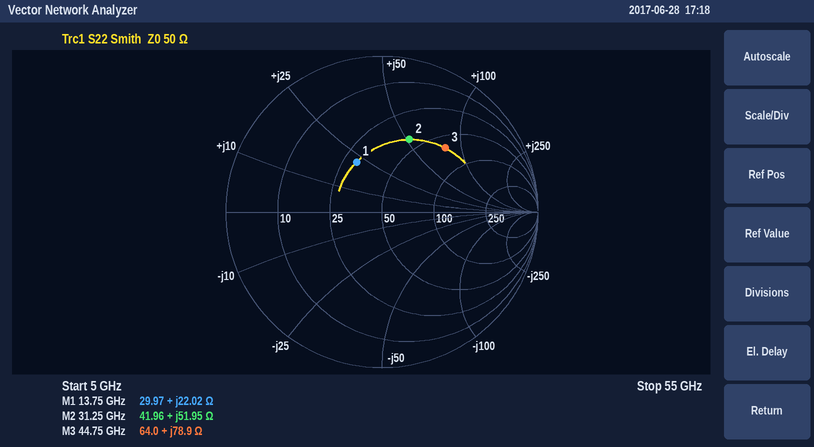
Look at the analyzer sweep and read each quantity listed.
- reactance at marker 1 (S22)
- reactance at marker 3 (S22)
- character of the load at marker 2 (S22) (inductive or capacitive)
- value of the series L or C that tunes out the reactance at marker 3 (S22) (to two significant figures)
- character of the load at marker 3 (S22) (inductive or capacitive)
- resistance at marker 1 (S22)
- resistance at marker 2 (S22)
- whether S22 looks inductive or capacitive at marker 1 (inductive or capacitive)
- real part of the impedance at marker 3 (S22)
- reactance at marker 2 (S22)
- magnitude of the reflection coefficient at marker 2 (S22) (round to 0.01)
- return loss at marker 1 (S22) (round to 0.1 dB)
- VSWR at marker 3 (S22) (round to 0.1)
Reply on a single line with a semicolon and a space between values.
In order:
+22.02 Ω; +78.9 Ω; inductive; 45 fF; inductive; 29.97 Ω; 41.96 Ω; inductive; 64.0 Ω; +51.95 Ω; 0.50; 8.9 dB; 3.7
